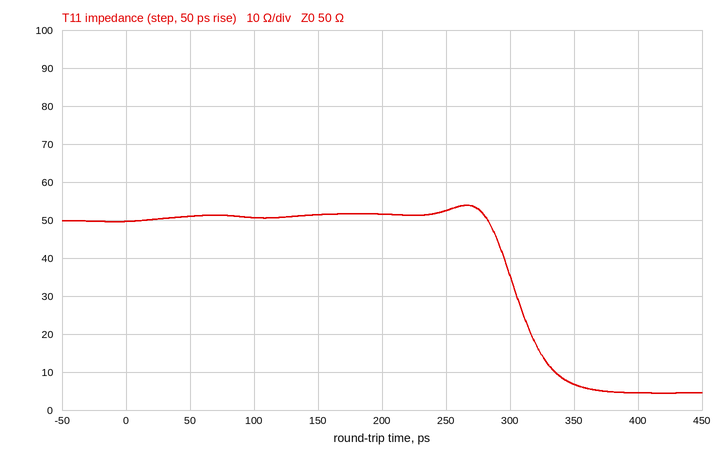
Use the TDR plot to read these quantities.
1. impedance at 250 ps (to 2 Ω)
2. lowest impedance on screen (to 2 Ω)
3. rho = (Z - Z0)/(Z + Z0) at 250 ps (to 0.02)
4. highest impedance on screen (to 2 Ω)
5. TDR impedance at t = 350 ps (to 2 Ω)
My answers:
52 Ω
4 Ω
+0.02
54 Ω
6 Ω
